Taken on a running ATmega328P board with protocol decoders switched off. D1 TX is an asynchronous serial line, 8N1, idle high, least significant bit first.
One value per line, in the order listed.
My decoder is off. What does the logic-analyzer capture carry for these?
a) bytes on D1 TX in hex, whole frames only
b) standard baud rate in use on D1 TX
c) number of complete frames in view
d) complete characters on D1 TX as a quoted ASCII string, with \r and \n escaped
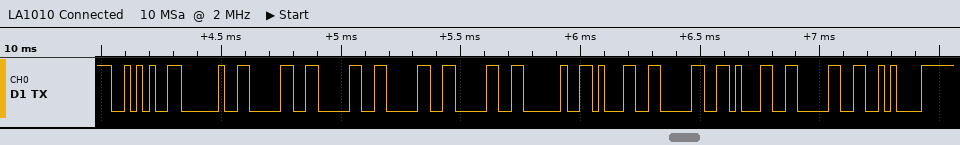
2A 20 30 30 30 30 20 31 30 31 30 0A
38400 baud
12
"* 0000 1010\n"
